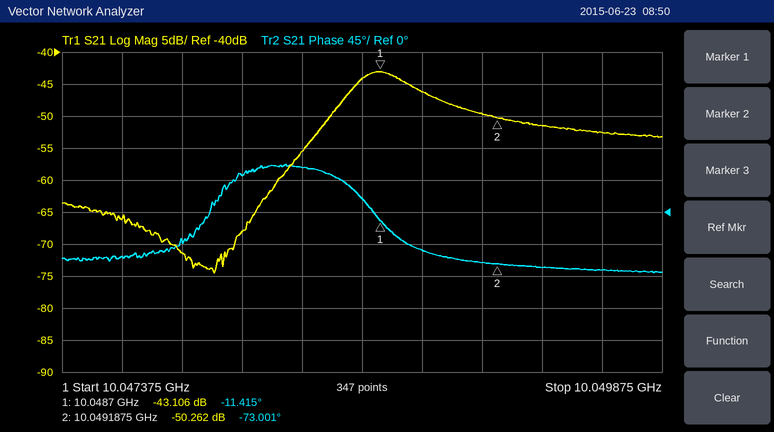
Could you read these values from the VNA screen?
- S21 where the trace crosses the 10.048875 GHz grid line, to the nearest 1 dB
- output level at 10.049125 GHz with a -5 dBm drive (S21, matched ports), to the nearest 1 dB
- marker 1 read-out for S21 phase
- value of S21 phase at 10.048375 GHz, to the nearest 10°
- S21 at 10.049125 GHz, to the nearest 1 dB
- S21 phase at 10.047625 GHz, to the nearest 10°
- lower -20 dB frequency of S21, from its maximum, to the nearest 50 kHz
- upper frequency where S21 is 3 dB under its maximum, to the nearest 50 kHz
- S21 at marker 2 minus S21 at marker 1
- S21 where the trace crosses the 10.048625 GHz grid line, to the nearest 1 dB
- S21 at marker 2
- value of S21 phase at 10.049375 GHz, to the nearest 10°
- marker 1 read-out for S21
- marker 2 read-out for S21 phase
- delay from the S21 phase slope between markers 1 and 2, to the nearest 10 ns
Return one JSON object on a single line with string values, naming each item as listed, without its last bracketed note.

{"S21 where the trace crosses the 10.048875 GHz grid line, to the nearest 1 dB": "-46 dB", "output level at 10.049125 GHz with a -5 dBm drive (S21, matched ports), to the nearest 1 dB": "-55 dBm", "marker 1 read-out for S21 phase": "-11.415°", "value of S21 phase at 10.048375 GHz, to the nearest 10°": "60°", "S21 at 10.049125 GHz, to the nearest 1 dB": "-50 dB", "S21 phase at 10.047625 GHz, to the nearest 10°": "-60°", "lower -20 dB frequency of S21, from its maximum, to the nearest 50 kHz": "10.04820 GHz", "upper frequency where S21 is 3 dB under its maximum, to the nearest 50 kHz": "10.04885 GHz", "S21 at marker 2 minus S21 at marker 1": "-7.156 dB", "S21 where the trace crosses the 10.048625 GHz grid line, to the nearest 1 dB": "-44 dB", "S21 at marker 2": "-50.262 dB", "value of S21 phase at 10.049375 GHz, to the nearest 10°": "-80°", "marker 1 read-out for S21": "-43.106 dB", "marker 2 read-out for S21 phase": "-73.001°", "delay from the S21 phase slope between markers 1 and 2, to the nearest 10 ns": "350 ns"}
